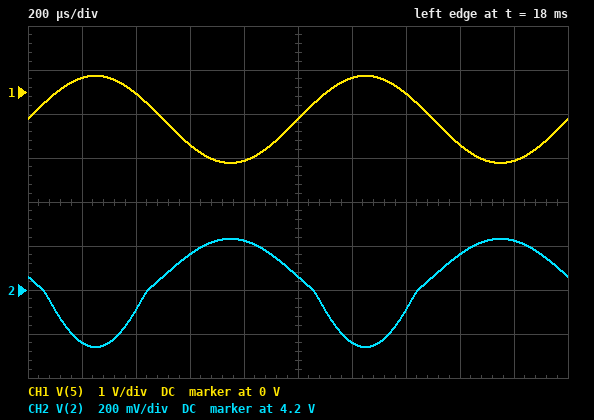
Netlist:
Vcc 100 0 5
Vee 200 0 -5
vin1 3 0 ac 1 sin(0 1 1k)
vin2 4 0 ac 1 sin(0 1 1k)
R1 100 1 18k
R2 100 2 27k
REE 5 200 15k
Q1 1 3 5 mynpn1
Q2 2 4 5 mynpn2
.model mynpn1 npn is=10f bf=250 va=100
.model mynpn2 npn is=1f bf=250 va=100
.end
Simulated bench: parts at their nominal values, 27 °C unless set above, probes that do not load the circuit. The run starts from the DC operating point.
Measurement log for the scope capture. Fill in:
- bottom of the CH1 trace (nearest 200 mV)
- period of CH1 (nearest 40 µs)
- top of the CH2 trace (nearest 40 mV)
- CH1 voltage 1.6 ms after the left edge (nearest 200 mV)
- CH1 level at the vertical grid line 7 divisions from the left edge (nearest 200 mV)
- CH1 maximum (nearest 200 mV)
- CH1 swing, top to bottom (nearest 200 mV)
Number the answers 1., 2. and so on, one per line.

1. -1.6 V
2. 1.00 ms
3. 4.44 V
4. -1.2 V
5. 0 V
6. 400 mV
7. 2.0 V
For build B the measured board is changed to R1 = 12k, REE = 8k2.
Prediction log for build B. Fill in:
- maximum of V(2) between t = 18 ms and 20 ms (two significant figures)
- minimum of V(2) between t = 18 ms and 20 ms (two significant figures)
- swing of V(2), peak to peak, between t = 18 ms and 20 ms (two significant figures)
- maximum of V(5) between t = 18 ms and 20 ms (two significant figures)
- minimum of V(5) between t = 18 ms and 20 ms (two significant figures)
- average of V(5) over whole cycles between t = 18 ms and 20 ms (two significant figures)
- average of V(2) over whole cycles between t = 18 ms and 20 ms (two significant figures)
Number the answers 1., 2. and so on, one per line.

1. 4.0 V
2. 2.9 V
3. 1.1 V
4. 350 mV
5. -1.6 V
6. -640 mV
7. 3.5 V
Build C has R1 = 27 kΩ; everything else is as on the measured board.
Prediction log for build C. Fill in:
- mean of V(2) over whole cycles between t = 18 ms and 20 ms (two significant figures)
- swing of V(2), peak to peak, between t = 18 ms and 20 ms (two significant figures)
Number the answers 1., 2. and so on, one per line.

1. 4.1 V
2. 670 mV
